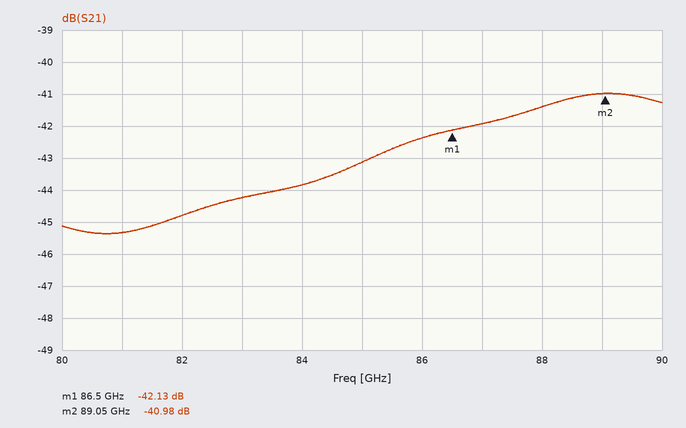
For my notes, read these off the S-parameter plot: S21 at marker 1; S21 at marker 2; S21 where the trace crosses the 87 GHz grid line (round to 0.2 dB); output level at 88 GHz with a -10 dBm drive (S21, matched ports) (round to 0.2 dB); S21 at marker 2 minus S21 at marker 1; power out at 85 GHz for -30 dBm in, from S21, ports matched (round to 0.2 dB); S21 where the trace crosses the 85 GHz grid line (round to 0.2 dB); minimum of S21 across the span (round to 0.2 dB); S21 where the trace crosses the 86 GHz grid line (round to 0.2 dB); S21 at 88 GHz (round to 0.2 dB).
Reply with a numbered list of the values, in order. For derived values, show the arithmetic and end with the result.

1. -42.13 dB
2. -40.98 dB
3. -42.0 dB
4. -10 dBm + (-41.4 dB) = -51.4 dBm
5. -40.98 − (-42.13) = 1.15 dB
6. -30 dBm + (-43.2 dB) = -73.2 dBm
7. -43.2 dB
8. -45.4 dB
9. -42.4 dB
10. -41.4 dB
